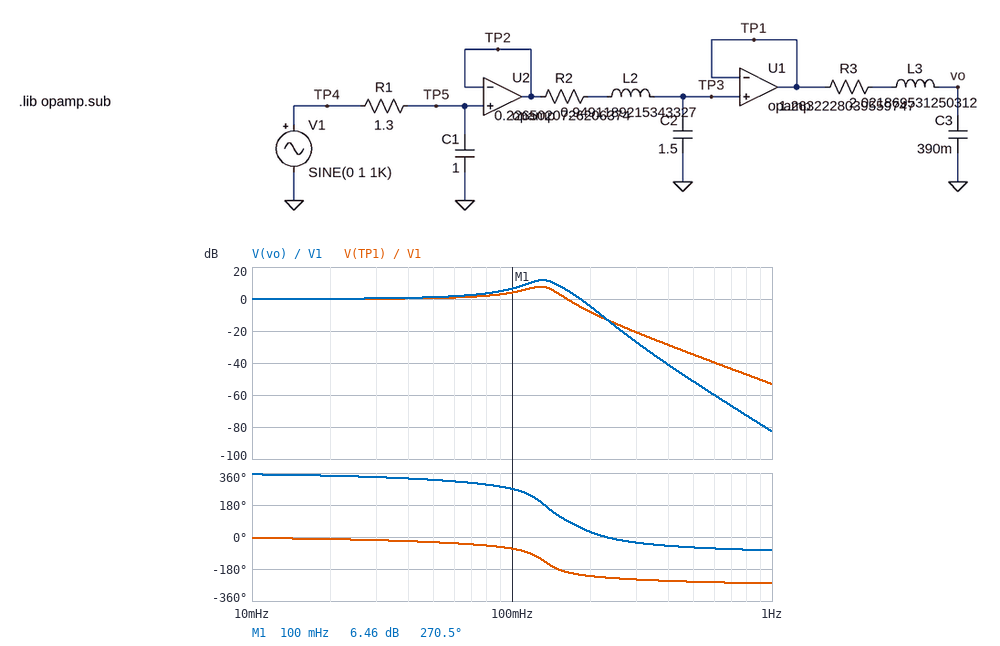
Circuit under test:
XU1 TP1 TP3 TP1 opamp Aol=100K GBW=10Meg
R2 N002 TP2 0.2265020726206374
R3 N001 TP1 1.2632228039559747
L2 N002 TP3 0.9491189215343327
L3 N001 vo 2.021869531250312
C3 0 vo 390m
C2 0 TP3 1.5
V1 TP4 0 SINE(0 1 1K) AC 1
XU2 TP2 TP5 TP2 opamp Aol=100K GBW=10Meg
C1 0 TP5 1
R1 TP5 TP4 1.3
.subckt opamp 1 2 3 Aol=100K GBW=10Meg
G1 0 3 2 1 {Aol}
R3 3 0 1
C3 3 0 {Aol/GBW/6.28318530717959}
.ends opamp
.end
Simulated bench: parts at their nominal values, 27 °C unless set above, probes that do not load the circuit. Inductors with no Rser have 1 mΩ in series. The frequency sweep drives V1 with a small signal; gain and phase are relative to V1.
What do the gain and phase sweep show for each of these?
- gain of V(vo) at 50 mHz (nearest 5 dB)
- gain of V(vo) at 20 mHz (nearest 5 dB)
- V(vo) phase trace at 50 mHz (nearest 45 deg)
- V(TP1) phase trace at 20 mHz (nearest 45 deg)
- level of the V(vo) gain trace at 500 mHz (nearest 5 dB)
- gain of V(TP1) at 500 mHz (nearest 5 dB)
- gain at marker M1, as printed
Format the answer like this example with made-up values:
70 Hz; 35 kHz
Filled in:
0 dB; 0 dB; 315 deg; 0 deg; -50 dB; -35 dB; 6.46 dB
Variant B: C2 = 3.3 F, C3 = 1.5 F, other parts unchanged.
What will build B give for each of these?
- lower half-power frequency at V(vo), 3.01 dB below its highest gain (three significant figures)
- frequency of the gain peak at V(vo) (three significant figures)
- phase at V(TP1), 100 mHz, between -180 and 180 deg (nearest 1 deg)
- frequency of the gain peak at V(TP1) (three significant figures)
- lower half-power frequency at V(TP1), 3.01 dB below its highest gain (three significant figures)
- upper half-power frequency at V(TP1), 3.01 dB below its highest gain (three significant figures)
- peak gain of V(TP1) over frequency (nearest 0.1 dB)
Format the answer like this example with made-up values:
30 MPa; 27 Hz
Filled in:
51.2 mHz; 80.8 mHz; -156 deg; 84.3 mHz; 58.0 mHz; 101 mHz; 5.9 dB
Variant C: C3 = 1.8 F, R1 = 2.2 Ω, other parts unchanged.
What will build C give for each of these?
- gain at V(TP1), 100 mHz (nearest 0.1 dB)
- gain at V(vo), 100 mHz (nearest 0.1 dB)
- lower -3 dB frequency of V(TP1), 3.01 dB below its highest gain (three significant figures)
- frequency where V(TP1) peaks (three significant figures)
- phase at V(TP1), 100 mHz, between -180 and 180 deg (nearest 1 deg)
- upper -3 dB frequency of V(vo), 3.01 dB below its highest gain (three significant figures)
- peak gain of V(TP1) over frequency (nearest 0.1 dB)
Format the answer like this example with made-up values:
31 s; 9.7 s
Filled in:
1.6 dB; -1.9 dB; 101 mHz; 128 mHz; -80 deg; 132 mHz; 4.7 dB
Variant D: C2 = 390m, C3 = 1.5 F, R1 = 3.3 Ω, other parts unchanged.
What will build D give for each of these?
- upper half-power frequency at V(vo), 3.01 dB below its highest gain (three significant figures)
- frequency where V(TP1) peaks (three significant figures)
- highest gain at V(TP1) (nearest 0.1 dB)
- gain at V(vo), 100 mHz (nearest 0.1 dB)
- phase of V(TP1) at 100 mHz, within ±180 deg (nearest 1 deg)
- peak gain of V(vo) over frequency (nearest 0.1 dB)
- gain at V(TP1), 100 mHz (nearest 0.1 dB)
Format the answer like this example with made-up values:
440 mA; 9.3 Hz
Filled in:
62.5 mHz; 259 mHz; 2.0 dB; -7.5 dB; -68 deg; 0 dB; -5.9 dB
